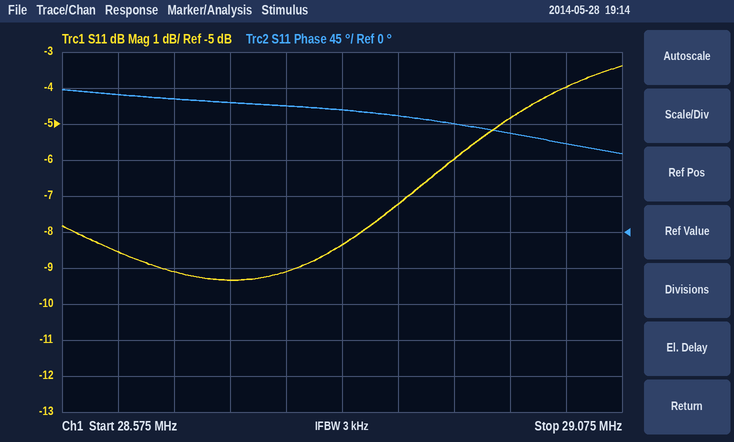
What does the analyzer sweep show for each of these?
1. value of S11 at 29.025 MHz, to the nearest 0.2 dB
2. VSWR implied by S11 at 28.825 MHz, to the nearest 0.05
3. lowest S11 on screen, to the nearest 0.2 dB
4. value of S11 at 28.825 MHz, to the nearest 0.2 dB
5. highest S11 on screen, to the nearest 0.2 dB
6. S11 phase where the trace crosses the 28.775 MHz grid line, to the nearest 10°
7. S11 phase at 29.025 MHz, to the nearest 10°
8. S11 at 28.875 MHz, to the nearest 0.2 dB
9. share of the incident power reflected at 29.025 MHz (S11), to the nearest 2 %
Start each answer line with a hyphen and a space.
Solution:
- -4.0 dB
- 2.25
- -9.4 dB
- -8.4 dB
- -3.4 dB
- 160°
- 110°
- -7.2 dB
- 40 %
